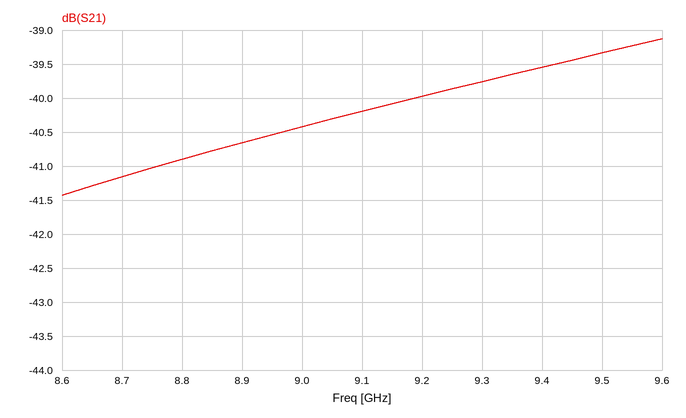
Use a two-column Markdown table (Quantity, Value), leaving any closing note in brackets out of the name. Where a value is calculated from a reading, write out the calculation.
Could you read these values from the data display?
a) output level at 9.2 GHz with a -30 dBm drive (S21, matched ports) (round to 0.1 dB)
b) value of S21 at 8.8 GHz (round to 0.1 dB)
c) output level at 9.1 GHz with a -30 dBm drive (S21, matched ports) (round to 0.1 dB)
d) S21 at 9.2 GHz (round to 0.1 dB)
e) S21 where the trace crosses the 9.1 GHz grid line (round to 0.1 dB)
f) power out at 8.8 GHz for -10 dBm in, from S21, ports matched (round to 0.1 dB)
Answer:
| Quantity | Value |
|---|---|
| output level at 9.2 GHz with a -30 dBm drive (S21, matched ports) | -30 dBm + (-40.0 dB) = -70.0 dBm |
| value of S21 at 8.8 GHz | -40.9 dB |
| output level at 9.1 GHz with a -30 dBm drive (S21, matched ports) | -30 dBm + (-40.2 dB) = -70.2 dBm |
| S21 at 9.2 GHz | -40.0 dB |
| S21 where the trace crosses the 9.1 GHz grid line | -40.2 dB |
| power out at 8.8 GHz for -10 dBm in, from S21, ports matched | -10 dBm + (-40.9 dB) = -50.9 dBm |
